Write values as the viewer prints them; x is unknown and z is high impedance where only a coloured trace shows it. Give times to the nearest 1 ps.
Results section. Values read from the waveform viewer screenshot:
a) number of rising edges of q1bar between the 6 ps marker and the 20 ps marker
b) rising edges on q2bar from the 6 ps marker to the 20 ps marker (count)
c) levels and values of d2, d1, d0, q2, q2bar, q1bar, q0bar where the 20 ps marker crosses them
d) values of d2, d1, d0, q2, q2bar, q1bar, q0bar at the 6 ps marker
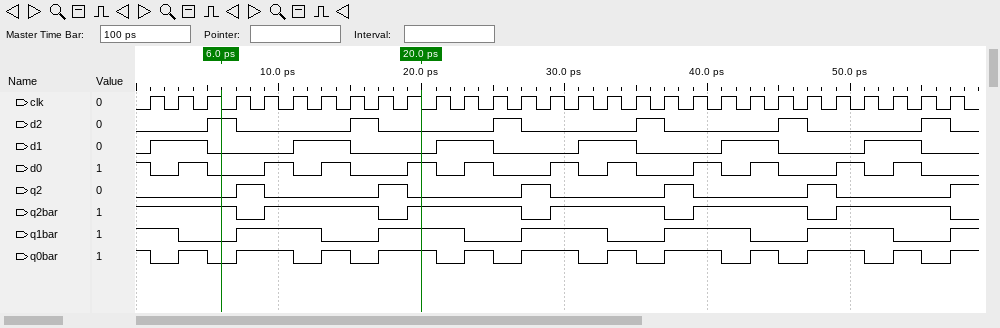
2
2
d2=0, d1=0, d0=1, q2=0, q2bar=1, q1bar=1, q0bar=1
d2=1, d1=0, d0=0, q2=0, q2bar=1, q1bar=0, q0bar=0
